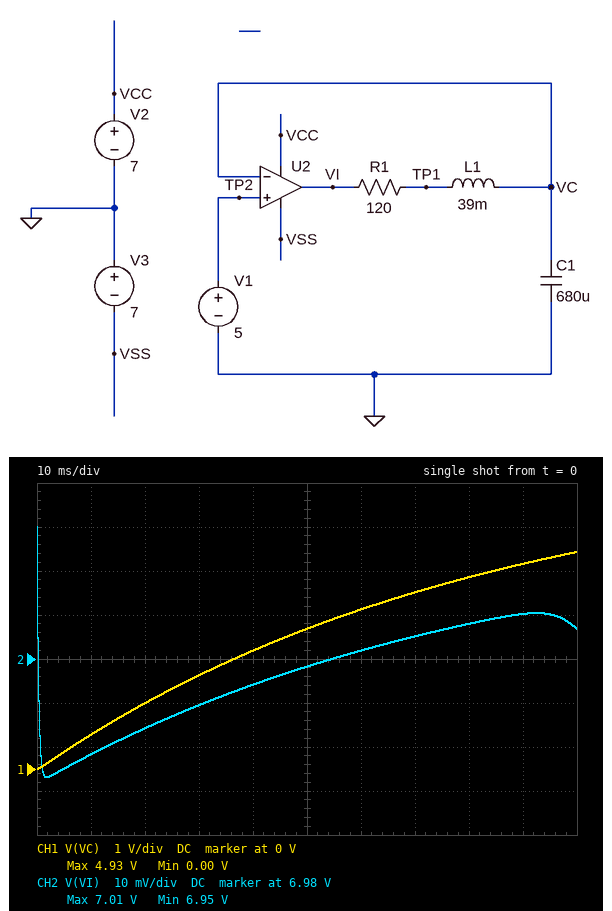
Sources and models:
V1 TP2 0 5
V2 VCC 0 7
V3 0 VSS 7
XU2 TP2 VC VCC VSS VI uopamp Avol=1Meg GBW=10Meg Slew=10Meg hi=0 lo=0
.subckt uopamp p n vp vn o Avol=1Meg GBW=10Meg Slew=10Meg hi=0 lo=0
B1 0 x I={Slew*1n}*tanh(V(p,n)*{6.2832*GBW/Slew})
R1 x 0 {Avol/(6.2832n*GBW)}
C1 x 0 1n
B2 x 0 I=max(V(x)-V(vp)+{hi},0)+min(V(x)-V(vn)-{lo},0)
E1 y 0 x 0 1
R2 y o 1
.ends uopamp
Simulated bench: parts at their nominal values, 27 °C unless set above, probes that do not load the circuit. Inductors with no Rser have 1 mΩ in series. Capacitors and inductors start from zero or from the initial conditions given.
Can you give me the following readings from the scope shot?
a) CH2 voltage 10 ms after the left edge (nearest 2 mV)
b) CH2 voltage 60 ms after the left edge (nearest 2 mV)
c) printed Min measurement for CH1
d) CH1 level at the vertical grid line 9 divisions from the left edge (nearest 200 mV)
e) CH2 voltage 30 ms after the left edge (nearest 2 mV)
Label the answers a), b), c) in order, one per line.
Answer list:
a) 6.958 V
b) 6.982 V
c) 0.00 V
d) 4.6 V
e) 6.970 V
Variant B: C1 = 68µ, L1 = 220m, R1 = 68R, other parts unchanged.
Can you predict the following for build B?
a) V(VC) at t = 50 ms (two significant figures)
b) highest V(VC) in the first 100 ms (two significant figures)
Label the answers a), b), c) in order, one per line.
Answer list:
a) 4.9 V
b) 5.3 V
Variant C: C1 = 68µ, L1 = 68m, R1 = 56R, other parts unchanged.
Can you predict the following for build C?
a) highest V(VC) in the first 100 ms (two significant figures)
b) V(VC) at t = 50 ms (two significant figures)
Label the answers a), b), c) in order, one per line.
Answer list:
a) 5.1 V
b) 5.0 V
